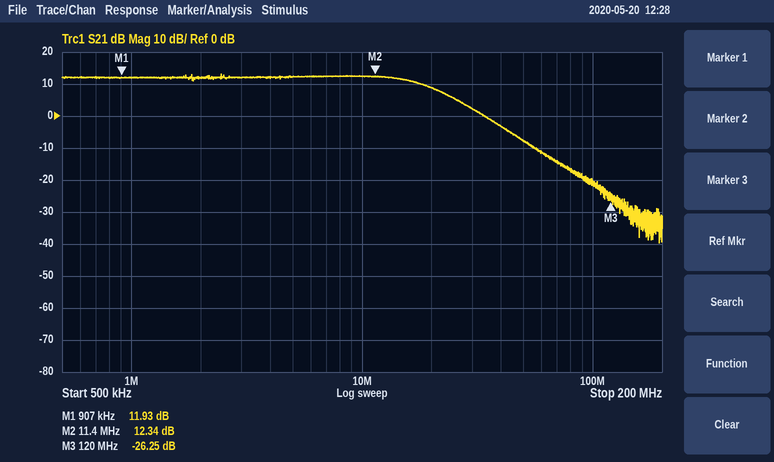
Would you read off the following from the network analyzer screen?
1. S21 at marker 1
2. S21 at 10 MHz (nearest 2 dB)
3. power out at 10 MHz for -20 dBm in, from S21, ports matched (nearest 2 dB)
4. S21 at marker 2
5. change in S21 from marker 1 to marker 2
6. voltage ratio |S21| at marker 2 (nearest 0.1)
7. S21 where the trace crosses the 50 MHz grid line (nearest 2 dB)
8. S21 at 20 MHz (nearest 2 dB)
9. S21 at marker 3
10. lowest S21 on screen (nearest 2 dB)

11.93 dB
12 dB
-8 dBm
12.34 dB
0.41 dB
4.1
-8 dB
8 dB
-26.25 dB
-40 dB
